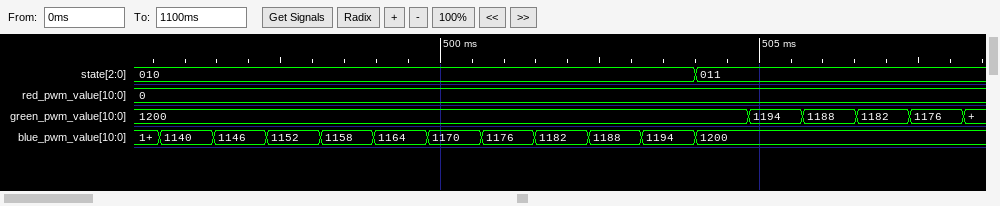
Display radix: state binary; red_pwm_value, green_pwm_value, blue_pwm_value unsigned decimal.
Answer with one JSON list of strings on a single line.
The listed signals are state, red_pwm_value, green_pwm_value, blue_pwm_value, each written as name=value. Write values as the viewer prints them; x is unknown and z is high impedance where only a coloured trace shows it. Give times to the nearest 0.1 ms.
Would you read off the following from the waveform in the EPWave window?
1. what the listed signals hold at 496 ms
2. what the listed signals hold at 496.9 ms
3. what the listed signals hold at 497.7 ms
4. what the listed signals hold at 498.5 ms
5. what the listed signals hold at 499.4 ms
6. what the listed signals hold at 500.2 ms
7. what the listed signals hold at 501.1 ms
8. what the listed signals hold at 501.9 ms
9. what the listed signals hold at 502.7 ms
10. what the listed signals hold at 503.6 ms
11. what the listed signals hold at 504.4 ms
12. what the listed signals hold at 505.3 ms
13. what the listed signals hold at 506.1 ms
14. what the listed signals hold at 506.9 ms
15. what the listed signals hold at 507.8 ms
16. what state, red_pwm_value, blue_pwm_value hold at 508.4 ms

["state=010, red_pwm_value=0, green_pwm_value=1200, blue_pwm_value=1140", "state=010, red_pwm_value=0, green_pwm_value=1200, blue_pwm_value=1146", "state=010, red_pwm_value=0, green_pwm_value=1200, blue_pwm_value=1152", "state=010, red_pwm_value=0, green_pwm_value=1200, blue_pwm_value=1158", "state=010, red_pwm_value=0, green_pwm_value=1200, blue_pwm_value=1164", "state=010, red_pwm_value=0, green_pwm_value=1200, blue_pwm_value=1170", "state=010, red_pwm_value=0, green_pwm_value=1200, blue_pwm_value=1176", "state=010, red_pwm_value=0, green_pwm_value=1200, blue_pwm_value=1182", "state=010, red_pwm_value=0, green_pwm_value=1200, blue_pwm_value=1188", "state=010, red_pwm_value=0, green_pwm_value=1200, blue_pwm_value=1194", "state=011, red_pwm_value=0, green_pwm_value=1200, blue_pwm_value=1200", "state=011, red_pwm_value=0, green_pwm_value=1194, blue_pwm_value=1200", "state=011, red_pwm_value=0, green_pwm_value=1188, blue_pwm_value=1200", "state=011, red_pwm_value=0, green_pwm_value=1182, blue_pwm_value=1200", "state=011, red_pwm_value=0, green_pwm_value=1176, blue_pwm_value=1200", "state=011, red_pwm_value=0, blue_pwm_value=1200"]
